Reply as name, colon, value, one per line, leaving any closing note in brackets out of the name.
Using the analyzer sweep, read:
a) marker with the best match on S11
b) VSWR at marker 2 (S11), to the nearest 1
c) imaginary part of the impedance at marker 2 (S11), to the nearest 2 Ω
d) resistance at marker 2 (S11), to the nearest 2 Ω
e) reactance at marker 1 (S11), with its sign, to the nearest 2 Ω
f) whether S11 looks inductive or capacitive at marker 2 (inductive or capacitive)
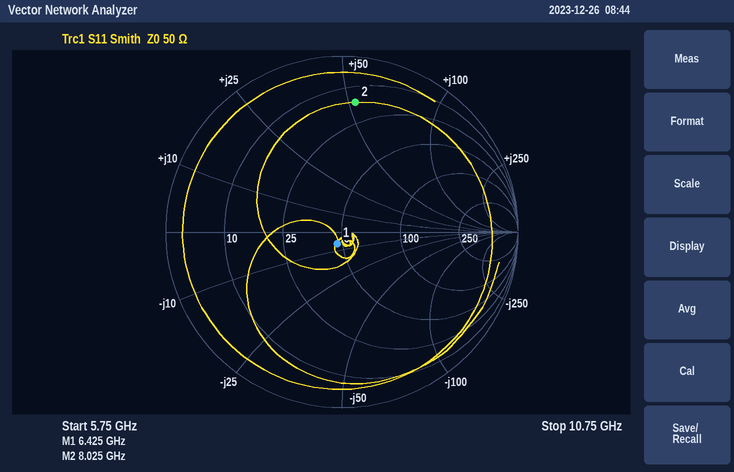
marker with the best match on S11: marker 1
VSWR at marker 2 (S11), to the nearest 1: 7
imaginary part of the impedance at marker 2 (S11), to the nearest 2 Ω: +52 Ω
resistance at marker 2 (S11), to the nearest 2 Ω: 16 Ω
reactance at marker 1 (S11), with its sign, to the nearest 2 Ω: -6 Ω
whether S11 looks inductive or capacitive at marker 2: inductive
